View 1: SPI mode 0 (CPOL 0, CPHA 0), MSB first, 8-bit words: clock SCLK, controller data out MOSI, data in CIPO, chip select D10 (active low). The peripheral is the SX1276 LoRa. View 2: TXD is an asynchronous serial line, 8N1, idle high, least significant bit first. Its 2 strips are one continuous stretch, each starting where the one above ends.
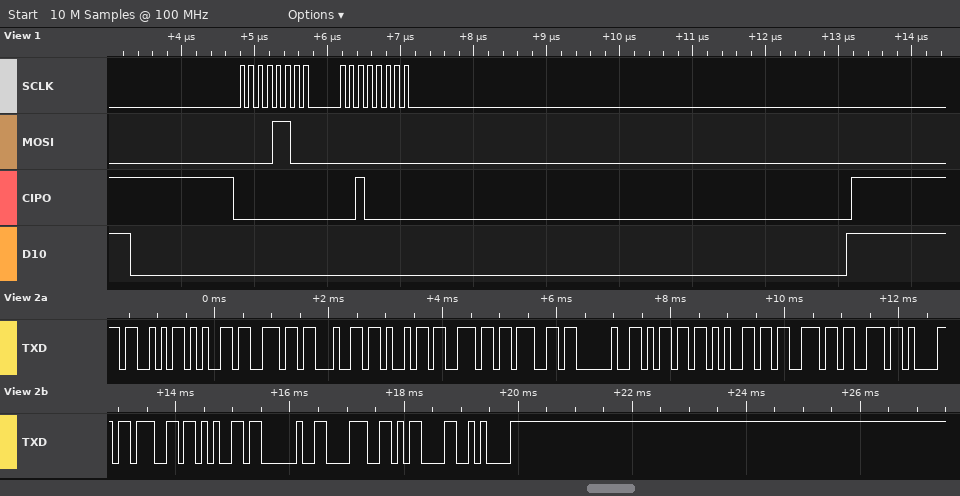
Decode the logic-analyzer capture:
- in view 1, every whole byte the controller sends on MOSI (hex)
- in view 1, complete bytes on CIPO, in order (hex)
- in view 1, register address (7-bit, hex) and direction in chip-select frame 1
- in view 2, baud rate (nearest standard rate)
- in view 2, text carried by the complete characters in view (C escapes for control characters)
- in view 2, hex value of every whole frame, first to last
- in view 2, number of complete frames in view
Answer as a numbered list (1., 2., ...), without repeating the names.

1. 0C 00
2. 00 20
3. 0x0C read
4. 9600 baud
5. "Sending message 8\r\n"
6. 53 65 6E 64 69 6E 67 20 6D 65 73 73 61 67 65 20 38 0D 0A
7. 19
